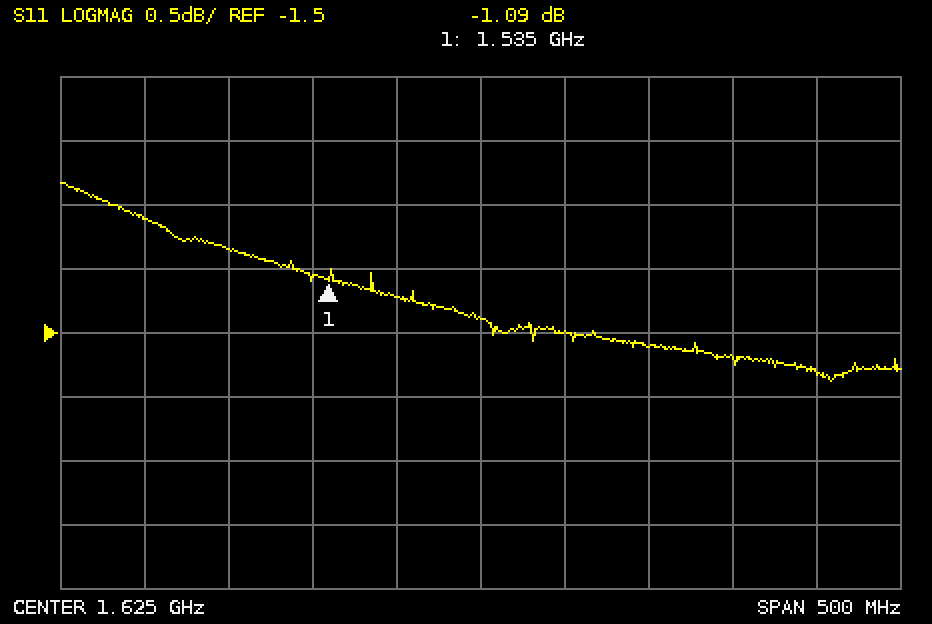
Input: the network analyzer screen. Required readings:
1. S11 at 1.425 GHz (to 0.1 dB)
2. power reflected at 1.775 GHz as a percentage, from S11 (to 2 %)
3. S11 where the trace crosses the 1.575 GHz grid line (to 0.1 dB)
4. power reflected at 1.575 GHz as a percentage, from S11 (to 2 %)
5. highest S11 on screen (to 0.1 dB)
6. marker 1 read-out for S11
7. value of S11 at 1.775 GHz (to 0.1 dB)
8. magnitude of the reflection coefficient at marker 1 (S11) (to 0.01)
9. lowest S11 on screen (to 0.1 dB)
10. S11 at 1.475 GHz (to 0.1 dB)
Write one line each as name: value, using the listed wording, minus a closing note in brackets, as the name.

S11 at 1.425 GHz: -0.6 dB
power reflected at 1.775 GHz as a percentage, from S11: 68 %
S11 where the trace crosses the 1.575 GHz grid line: -1.2 dB
power reflected at 1.575 GHz as a percentage, from S11: 76 %
highest S11 on screen: -0.3 dB
marker 1 read-out for S11: -1.09 dB
value of S11 at 1.775 GHz: -1.7 dB
magnitude of the reflection coefficient at marker 1 (S11): 0.88
lowest S11 on screen: -1.9 dB
S11 at 1.475 GHz: -0.8 dB
